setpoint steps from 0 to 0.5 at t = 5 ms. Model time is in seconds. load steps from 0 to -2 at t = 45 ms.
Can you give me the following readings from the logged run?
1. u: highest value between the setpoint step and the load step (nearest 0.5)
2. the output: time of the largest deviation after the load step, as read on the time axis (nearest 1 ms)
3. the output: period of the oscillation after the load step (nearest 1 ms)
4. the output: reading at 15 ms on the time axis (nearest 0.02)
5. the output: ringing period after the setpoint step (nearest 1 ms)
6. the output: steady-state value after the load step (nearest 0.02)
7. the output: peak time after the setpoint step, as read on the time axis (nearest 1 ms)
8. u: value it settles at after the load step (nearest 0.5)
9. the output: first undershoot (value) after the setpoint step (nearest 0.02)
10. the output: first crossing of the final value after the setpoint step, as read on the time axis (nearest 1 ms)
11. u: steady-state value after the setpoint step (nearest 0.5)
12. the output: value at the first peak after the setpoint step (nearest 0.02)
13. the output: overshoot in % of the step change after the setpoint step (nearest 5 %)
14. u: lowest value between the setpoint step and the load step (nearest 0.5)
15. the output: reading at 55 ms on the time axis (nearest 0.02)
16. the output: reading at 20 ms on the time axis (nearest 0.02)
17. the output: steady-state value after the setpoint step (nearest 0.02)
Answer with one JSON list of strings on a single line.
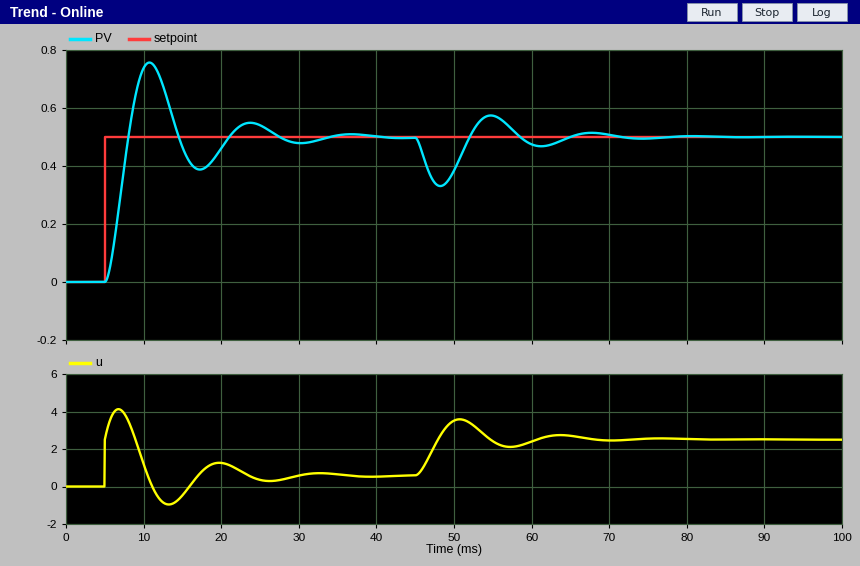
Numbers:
["4.0", "48 ms", "13 ms", "0.46", "13 ms", "0.50", "11 ms", "2.5", "0.38", "8 ms", "0.5", "0.76", "50 %", "-1.0", "0.58", "0.46", "0.50"]
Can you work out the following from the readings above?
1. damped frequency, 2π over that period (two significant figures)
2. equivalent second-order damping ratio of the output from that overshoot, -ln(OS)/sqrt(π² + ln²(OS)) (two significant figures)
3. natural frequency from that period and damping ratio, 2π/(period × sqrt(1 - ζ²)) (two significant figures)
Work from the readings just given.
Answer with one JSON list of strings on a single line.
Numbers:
["0.48 rad/ms", "0.22", "0.50 rad/ms"]
